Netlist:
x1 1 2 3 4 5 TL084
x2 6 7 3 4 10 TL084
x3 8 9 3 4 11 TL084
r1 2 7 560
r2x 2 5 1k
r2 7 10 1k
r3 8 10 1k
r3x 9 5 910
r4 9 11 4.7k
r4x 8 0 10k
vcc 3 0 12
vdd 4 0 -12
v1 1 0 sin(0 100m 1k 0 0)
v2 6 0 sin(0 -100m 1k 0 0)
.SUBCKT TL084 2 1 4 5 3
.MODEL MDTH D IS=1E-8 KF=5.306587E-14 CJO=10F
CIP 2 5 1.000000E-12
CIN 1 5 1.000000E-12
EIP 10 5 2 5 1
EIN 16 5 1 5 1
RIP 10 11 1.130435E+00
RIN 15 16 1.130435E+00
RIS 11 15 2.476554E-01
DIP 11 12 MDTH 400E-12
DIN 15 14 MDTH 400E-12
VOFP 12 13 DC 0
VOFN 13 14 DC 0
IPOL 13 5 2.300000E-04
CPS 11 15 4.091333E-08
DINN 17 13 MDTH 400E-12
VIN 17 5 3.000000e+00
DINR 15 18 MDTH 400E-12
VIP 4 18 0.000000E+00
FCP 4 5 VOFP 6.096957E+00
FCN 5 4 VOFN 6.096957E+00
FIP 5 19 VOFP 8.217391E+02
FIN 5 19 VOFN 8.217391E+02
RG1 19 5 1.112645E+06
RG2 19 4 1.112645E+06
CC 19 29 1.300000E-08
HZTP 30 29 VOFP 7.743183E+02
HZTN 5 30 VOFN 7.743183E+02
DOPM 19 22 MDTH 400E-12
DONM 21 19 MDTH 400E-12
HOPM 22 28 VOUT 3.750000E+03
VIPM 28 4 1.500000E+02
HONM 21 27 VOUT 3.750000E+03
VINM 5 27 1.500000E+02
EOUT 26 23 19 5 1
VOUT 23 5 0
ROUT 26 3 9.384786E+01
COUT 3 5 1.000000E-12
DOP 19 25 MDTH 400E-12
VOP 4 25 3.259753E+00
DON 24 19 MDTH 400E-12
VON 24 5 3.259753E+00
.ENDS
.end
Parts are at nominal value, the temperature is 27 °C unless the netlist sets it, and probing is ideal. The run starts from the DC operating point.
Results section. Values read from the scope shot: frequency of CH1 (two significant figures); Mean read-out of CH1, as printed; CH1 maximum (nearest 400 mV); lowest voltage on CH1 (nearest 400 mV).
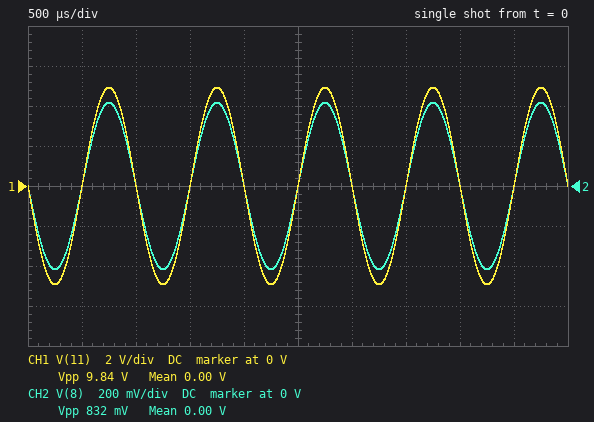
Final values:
1.0 kHz
0.00 V
4.8 V
-4.8 V
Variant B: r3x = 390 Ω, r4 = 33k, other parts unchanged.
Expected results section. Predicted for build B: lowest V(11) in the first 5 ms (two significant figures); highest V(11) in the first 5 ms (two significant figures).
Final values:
-9.7 V
9.7 V
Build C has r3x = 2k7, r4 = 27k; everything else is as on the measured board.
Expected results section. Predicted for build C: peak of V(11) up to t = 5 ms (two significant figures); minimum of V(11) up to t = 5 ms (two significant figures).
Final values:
9.1 V
-9.1 V
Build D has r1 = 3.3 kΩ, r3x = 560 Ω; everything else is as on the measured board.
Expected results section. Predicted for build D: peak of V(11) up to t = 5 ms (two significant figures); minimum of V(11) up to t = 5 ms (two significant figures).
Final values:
2.7 V
-2.7 V
